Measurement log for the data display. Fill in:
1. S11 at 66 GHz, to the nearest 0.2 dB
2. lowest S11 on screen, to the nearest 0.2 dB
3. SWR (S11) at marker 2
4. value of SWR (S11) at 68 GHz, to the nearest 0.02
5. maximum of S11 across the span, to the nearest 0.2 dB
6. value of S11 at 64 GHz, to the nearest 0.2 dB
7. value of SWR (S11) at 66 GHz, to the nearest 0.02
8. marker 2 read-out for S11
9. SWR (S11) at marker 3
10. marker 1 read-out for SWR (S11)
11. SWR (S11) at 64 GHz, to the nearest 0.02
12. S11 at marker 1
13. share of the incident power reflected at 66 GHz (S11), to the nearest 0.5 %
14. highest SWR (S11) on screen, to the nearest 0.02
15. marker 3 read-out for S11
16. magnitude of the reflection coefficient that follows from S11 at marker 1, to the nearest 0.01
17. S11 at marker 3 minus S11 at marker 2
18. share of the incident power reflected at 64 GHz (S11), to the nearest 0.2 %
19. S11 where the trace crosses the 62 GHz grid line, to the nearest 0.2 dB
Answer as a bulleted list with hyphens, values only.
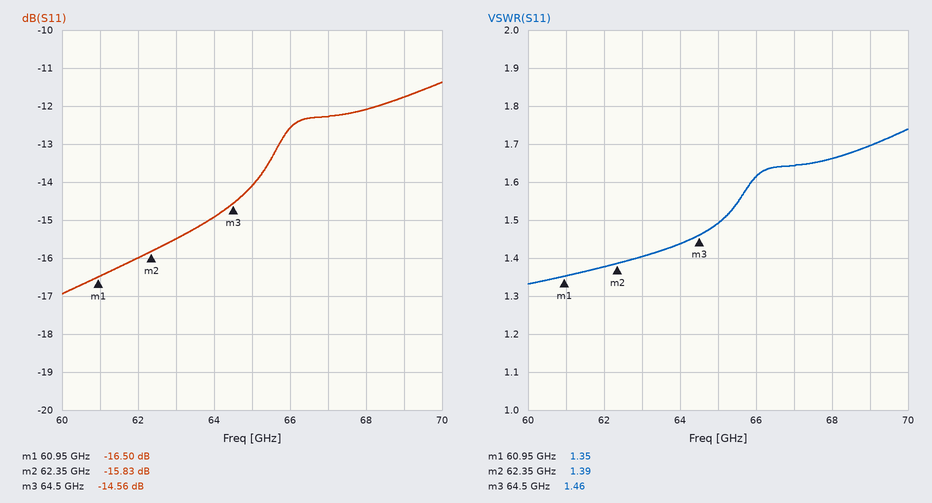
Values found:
- -12.6 dB
- -17.0 dB
- 1.39
- 1.66
- -11.4 dB
- -15.0 dB
- 1.62
- -15.83 dB
- 1.46
- 1.35
- 1.44
- -16.50 dB
- 5.5 %
- 1.74
- -14.56 dB
- 0.15
- 1.27 dB
- 3.2 %
- -16.0 dB
